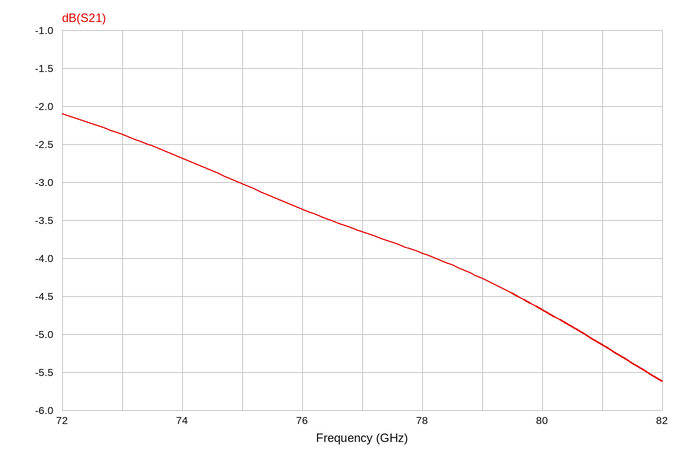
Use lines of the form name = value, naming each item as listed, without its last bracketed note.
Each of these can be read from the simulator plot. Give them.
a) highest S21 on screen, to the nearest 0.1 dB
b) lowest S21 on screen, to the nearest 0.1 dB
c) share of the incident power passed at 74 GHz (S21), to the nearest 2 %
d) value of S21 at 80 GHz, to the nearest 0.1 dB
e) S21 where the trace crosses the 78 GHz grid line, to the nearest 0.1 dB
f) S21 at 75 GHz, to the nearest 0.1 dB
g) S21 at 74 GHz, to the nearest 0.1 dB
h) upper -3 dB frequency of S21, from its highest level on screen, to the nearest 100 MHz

highest S21 on screen, to the nearest 0.1 dB = -2.1 dB
lowest S21 on screen, to the nearest 0.1 dB = -5.6 dB
share of the incident power passed at 74 GHz (S21), to the nearest 2 % = 54 %
value of S21 at 80 GHz, to the nearest 0.1 dB = -4.7 dB
S21 where the trace crosses the 78 GHz grid line, to the nearest 0.1 dB = -3.9 dB
S21 at 75 GHz, to the nearest 0.1 dB = -3.0 dB
S21 at 74 GHz, to the nearest 0.1 dB = -2.7 dB
upper -3 dB frequency of S21, from its highest level on screen, to the nearest 100 MHz = 80.9 GHz
